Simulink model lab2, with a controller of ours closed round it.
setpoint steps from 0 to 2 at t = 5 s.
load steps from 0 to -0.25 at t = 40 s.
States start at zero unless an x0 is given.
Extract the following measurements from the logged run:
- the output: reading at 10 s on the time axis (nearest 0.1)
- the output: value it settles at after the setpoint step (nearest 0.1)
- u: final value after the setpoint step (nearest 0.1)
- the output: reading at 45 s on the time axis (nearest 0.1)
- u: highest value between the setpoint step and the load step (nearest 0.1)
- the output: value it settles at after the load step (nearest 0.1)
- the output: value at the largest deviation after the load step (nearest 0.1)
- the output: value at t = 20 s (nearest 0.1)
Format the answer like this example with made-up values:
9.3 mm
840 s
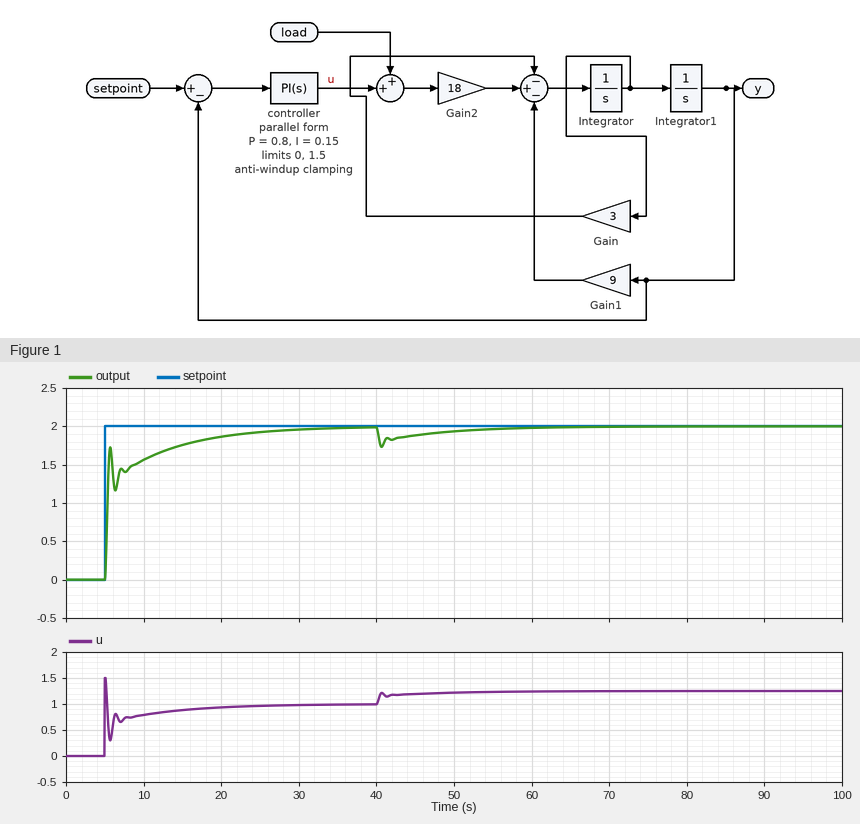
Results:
1.6
2.0
1.0
1.9
1.5
2.0
1.7
1.9
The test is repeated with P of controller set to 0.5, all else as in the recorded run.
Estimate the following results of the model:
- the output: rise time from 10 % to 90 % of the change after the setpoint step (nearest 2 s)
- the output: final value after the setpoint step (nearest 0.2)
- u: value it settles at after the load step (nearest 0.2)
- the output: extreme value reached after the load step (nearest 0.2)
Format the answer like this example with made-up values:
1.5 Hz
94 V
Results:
10 s
2.0
1.2
1.6
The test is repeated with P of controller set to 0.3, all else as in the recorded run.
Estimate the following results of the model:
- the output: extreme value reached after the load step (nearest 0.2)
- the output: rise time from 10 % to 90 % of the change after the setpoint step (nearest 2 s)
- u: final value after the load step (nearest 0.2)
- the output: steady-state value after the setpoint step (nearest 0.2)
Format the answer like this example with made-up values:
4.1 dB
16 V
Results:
1.6
10 s
1.2
2.0
